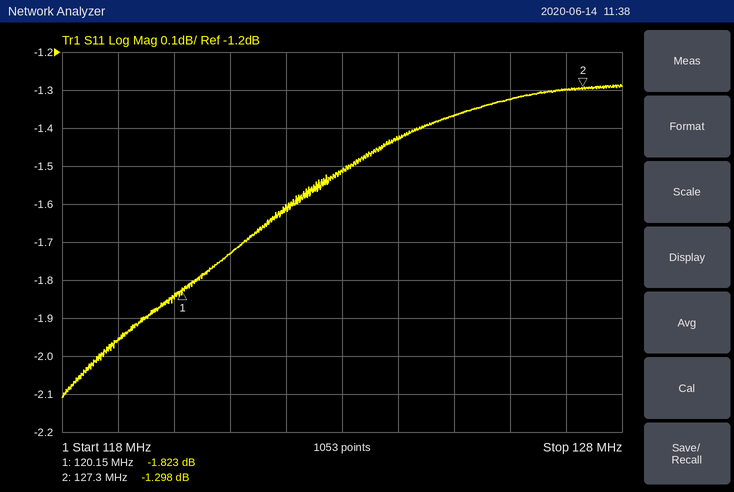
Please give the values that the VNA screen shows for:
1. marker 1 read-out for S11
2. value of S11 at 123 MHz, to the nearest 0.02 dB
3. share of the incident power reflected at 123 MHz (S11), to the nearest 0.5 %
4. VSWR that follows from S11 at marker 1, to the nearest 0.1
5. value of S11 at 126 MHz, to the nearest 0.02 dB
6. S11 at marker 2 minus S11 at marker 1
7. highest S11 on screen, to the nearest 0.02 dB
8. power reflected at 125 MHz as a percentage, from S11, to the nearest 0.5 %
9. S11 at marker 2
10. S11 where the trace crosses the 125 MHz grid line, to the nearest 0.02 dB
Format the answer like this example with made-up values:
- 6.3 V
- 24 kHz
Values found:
- -1.823 dB
- -1.52 dB
- 70.5 %
- 9.6
- -1.32 dB
- 0.525 dB
- -1.28 dB
- 73.0 %
- -1.298 dB
- -1.36 dB
